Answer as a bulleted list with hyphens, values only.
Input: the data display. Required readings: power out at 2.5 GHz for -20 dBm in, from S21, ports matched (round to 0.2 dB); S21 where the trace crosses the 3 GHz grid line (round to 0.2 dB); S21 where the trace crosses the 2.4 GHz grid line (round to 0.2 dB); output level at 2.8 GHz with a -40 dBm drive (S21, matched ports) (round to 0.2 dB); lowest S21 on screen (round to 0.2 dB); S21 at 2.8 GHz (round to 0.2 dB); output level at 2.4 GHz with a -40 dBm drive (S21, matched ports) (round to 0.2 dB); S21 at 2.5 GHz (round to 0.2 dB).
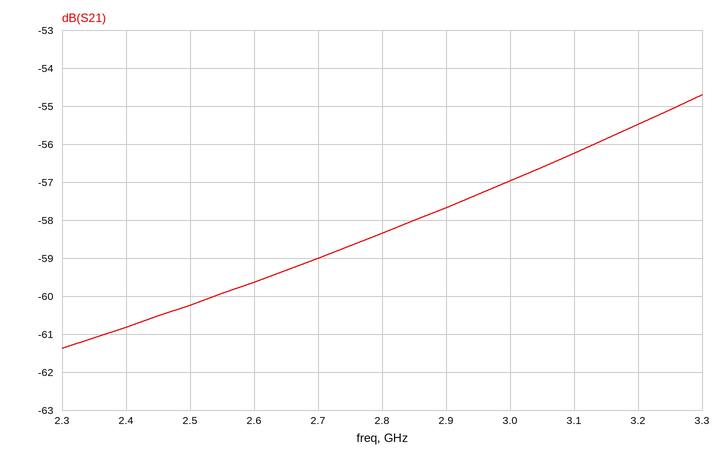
- -80.2 dBm
- -57.0 dB
- -60.8 dB
- -98.4 dBm
- -61.4 dB
- -58.4 dB
- -100.8 dBm
- -60.2 dB
